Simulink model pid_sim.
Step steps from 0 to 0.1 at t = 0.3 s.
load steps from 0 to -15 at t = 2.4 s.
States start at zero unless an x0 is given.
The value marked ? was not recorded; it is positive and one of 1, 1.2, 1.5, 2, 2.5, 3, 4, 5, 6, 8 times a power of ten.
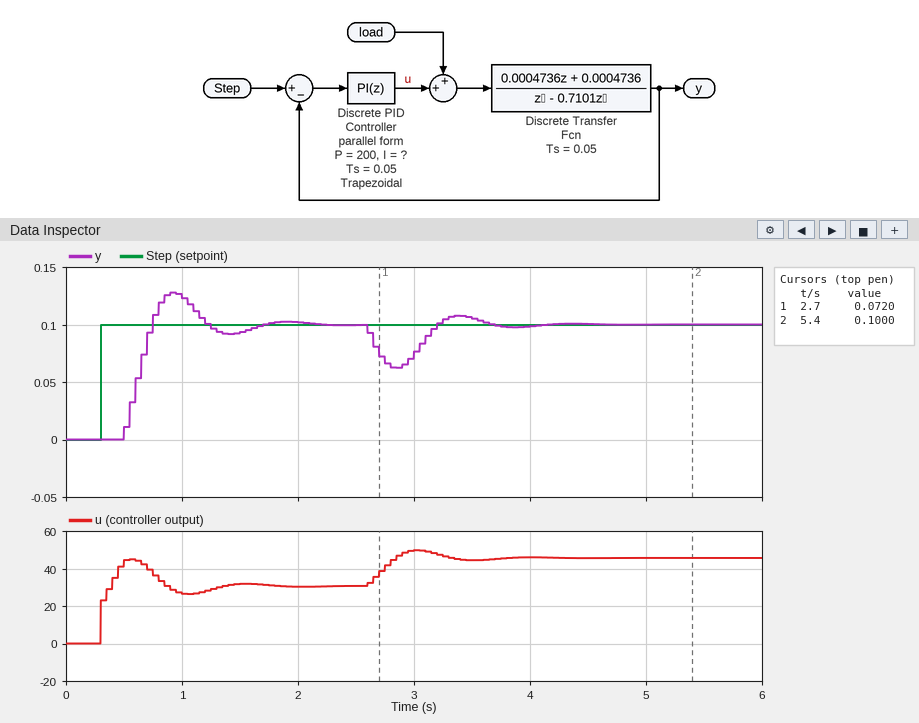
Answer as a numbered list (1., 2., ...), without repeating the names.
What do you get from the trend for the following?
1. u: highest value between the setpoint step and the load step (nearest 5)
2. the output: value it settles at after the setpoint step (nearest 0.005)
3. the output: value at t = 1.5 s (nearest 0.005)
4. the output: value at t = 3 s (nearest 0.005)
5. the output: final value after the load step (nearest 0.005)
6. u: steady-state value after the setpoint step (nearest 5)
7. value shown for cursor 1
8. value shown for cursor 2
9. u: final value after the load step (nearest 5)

1. 45
2. 0.100
3. 0.095
4. 0.075
5. 0.100
6. 30
7. 0.0720
8. 0.1000
9. 45
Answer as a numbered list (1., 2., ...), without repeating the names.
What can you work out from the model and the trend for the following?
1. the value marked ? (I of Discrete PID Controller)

1. 1200
